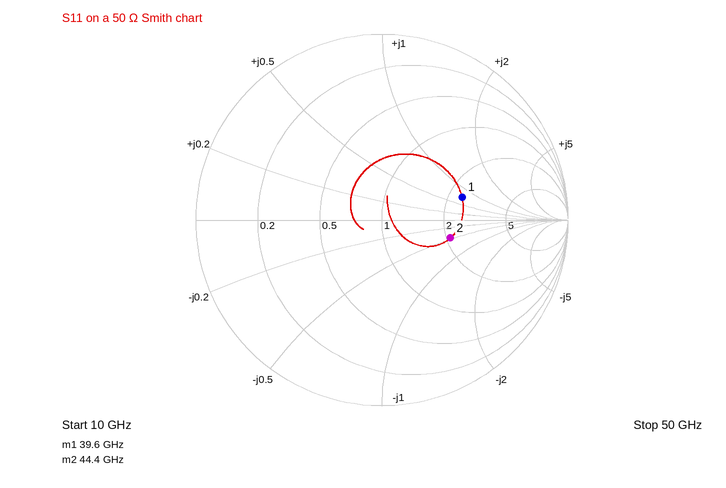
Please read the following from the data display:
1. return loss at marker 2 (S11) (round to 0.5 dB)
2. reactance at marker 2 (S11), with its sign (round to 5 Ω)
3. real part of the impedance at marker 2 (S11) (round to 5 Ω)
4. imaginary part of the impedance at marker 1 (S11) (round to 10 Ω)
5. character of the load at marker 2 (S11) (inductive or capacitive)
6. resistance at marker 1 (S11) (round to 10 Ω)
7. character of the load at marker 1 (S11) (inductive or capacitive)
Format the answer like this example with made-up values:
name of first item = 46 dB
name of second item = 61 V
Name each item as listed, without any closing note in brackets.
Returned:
return loss at marker 2 (S11) = 8.5 dB
reactance at marker 2 (S11), with its sign = -25 Ω
real part of the impedance at marker 2 (S11) = 105 Ω
imaginary part of the impedance at marker 1 (S11) = +40 Ω
character of the load at marker 2 (S11) = capacitive
resistance at marker 1 (S11) = 120 Ω
character of the load at marker 1 (S11) = inductive
